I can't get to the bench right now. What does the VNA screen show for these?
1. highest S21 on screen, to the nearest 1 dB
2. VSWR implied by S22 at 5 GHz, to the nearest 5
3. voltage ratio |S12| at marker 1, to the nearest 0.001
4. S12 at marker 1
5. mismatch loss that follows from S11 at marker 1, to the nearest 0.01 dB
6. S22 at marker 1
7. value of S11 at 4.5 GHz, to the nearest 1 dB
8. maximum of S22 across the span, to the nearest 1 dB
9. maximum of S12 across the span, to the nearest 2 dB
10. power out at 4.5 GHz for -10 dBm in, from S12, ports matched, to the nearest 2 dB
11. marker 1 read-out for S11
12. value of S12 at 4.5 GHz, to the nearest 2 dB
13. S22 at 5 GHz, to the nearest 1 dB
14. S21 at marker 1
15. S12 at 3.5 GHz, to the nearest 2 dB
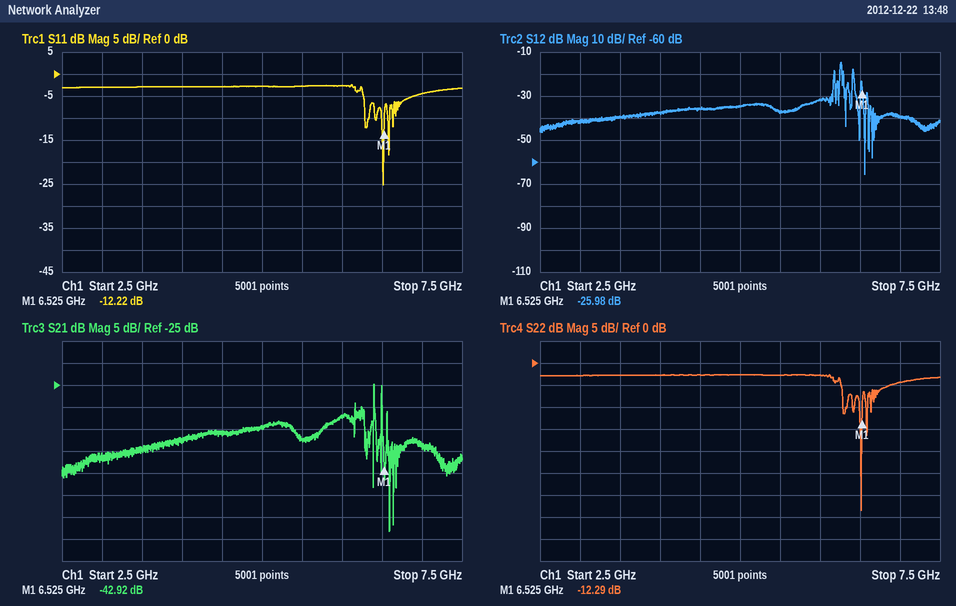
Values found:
-25 dB
5
0.050
-25.98 dB
0.27 dB
-12.29 dB
-3 dB
-3 dB
-14 dB
-46 dBm
-12.22 dB
-36 dB
-3 dB
-42.92 dB
-40 dB
